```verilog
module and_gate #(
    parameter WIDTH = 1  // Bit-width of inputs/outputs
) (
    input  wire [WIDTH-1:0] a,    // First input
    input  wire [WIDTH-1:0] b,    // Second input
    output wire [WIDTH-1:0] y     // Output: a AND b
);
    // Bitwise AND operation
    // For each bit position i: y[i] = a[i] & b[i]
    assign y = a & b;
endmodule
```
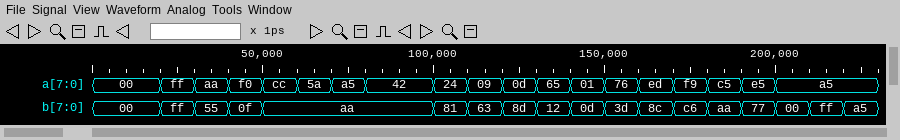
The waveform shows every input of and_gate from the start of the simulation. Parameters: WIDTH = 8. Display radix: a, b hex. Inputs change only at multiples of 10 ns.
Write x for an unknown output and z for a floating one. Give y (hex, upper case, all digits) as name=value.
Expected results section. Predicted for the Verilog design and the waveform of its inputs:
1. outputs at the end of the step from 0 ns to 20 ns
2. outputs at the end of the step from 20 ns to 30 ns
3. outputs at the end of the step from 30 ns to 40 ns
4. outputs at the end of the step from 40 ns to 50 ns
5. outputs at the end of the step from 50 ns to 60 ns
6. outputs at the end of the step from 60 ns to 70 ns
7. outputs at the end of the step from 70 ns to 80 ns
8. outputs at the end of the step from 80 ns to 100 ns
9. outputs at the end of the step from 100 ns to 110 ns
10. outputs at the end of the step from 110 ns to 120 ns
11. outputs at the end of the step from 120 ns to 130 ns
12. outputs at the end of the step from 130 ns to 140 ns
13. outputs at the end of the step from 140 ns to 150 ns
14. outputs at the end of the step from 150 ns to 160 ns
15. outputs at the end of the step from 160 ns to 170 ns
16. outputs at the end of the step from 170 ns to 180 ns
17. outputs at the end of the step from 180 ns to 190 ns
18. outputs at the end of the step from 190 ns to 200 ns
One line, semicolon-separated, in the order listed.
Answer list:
y=00; y=FF; y=00; y=00; y=88; y=0A; y=A0; y=02; y=00; y=01; y=0D; y=00; y=01; y=34; y=8C; y=C0; y=80; y=65
